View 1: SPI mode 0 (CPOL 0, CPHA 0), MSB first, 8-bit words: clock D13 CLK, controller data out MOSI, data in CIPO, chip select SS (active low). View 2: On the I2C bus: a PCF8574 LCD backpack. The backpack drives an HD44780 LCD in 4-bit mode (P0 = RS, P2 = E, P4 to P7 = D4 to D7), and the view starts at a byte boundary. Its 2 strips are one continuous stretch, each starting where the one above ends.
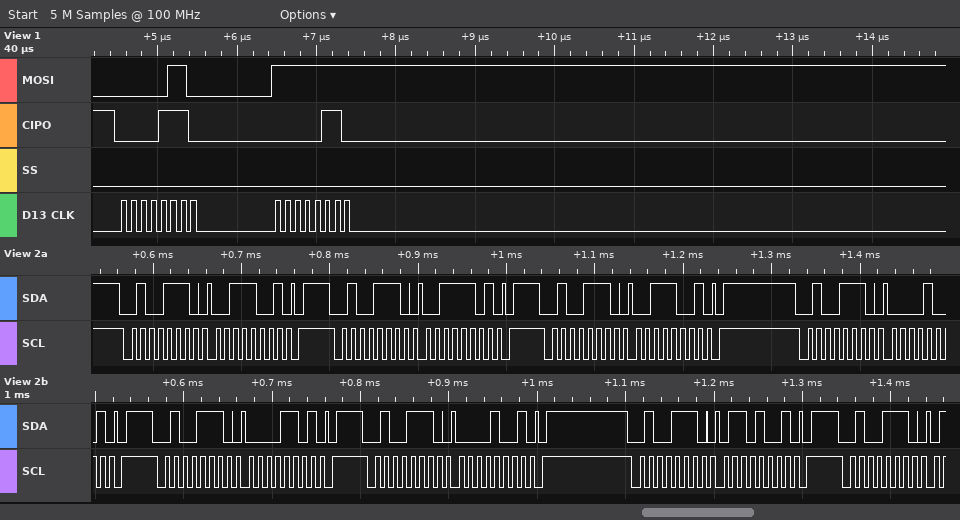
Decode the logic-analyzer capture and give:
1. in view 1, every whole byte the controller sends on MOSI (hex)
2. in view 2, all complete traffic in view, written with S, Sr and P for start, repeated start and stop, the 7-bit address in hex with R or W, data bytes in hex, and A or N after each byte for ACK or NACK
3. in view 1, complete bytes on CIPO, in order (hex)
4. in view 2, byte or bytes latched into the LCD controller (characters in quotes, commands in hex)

0x06 0xFF
S 27W A 39 A P S 27W A 3D A P S 27W A 39 A P S 27W A 09 A P S 27W A 0D A P S 27W A 09 A P S 27W A 69 A P S 27W A
0x0E 0x06
'0'
